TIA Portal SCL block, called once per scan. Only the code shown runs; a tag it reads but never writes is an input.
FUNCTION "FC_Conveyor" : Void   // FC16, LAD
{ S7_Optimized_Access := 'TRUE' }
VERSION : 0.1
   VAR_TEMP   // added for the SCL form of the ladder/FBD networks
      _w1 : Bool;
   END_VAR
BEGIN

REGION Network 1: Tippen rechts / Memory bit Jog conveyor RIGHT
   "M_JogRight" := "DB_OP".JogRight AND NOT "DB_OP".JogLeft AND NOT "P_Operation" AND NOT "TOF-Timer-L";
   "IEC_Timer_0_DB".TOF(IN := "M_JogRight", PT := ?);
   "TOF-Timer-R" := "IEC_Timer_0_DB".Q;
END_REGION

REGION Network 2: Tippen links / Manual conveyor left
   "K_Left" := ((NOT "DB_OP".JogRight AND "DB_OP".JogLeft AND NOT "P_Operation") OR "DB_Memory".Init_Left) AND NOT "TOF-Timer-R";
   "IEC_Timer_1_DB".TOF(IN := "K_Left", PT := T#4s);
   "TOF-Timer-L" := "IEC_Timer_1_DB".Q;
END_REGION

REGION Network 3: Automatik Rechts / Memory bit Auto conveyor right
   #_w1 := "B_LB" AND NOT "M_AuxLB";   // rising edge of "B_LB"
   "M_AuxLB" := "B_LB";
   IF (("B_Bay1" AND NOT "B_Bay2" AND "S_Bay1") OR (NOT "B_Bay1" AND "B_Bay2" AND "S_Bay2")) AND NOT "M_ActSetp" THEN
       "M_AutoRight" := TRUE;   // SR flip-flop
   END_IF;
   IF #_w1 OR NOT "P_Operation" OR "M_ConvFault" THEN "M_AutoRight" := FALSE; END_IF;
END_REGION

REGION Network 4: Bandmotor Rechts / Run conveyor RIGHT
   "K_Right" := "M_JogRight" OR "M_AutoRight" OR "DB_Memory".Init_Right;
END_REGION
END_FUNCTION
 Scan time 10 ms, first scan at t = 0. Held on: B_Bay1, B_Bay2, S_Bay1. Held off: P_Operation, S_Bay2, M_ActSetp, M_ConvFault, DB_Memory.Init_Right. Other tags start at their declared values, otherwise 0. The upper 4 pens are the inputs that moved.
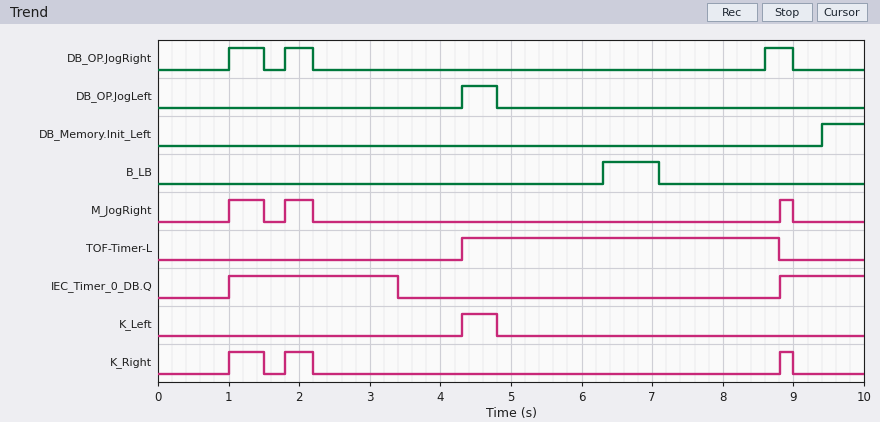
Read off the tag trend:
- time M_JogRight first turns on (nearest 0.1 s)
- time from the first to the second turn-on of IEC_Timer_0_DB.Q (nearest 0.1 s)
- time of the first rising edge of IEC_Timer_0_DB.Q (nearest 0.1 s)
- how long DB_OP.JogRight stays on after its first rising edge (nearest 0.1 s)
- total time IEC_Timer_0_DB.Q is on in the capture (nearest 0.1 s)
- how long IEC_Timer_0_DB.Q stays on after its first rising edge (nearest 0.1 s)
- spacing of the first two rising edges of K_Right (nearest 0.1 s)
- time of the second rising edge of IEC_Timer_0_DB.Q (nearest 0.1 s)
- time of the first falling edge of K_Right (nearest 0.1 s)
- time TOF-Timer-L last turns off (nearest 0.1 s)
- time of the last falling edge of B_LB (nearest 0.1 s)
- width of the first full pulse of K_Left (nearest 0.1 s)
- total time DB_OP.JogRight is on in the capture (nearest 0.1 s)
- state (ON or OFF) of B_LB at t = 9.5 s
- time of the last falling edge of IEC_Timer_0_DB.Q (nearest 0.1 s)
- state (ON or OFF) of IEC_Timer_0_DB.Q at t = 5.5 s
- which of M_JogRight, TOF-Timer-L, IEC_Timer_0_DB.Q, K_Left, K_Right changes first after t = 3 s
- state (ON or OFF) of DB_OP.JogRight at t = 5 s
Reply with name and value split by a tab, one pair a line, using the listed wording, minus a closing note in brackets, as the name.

time M_JogRight first turns on	1.0 s
time from the first to the second turn-on of IEC_Timer_0_DB.Q	7.8 s
time of the first rising edge of IEC_Timer_0_DB.Q	1.0 s
how long DB_OP.JogRight stays on after its first rising edge	0.5 s
total time IEC_Timer_0_DB.Q is on in the capture	3.6 s
how long IEC_Timer_0_DB.Q stays on after its first rising edge	2.4 s
spacing of the first two rising edges of K_Right	0.8 s
time of the second rising edge of IEC_Timer_0_DB.Q	8.8 s
time of the first falling edge of K_Right	1.5 s
time TOF-Timer-L last turns off	8.8 s
time of the last falling edge of B_LB	7.1 s
width of the first full pulse of K_Left	0.5 s
total time DB_OP.JogRight is on in the capture	1.3 s
state (ON or OFF) of B_LB at t = 9.5 s	OFF
time of the last falling edge of IEC_Timer_0_DB.Q	3.4 s
state (ON or OFF) of IEC_Timer_0_DB.Q at t = 5.5 s	OFF
which of M_JogRight, TOF-Timer-L, IEC_Timer_0_DB.Q, K_Left, K_Right changes first after t = 3 s	IEC_Timer_0_DB.Q
state (ON or OFF) of DB_OP.JogRight at t = 5 s	OFF
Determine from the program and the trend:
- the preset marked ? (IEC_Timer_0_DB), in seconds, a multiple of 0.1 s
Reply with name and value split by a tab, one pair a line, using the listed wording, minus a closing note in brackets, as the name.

the preset marked ? (IEC_Timer_0_DB), in seconds, a multiple of 0.1 s	1.2 s
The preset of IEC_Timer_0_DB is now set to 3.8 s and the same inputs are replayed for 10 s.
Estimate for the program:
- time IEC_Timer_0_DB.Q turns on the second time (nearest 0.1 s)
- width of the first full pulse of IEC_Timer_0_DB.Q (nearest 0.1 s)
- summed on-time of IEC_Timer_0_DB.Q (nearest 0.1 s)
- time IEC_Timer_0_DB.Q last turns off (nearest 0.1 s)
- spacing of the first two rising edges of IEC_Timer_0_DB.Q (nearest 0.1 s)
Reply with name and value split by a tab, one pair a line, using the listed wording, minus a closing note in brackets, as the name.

time IEC_Timer_0_DB.Q turns on the second time	8.6 s
width of the first full pulse of IEC_Timer_0_DB.Q	5.0 s
summed on-time of IEC_Timer_0_DB.Q	6.4 s
time IEC_Timer_0_DB.Q last turns off	6.0 s
spacing of the first two rising edges of IEC_Timer_0_DB.Q	7.6 s
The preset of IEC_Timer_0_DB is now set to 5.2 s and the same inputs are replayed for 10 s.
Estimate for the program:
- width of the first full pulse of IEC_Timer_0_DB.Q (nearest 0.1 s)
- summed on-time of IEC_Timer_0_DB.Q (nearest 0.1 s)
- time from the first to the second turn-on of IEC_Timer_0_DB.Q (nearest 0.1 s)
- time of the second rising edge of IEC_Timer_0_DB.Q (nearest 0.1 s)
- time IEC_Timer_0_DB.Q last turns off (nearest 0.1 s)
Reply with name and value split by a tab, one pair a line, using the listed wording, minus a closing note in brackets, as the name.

width of the first full pulse of IEC_Timer_0_DB.Q	6.4 s
summed on-time of IEC_Timer_0_DB.Q	7.8 s
time from the first to the second turn-on of IEC_Timer_0_DB.Q	7.6 s
time of the second rising edge of IEC_Timer_0_DB.Q	8.6 s
time IEC_Timer_0_DB.Q last turns off	7.4 s
